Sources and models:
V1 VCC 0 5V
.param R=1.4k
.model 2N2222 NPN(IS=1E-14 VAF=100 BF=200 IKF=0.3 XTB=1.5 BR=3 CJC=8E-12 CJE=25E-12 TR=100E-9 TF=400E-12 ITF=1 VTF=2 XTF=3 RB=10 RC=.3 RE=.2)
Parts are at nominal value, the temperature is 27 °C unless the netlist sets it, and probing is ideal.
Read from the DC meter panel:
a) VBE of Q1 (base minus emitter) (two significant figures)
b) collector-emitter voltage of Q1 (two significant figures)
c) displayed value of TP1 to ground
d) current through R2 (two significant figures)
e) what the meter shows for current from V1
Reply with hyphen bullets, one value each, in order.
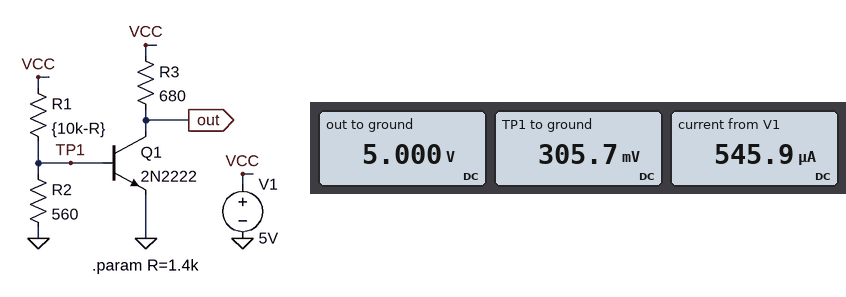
- 310 mV
- 5.0 V
- 305.7 mV
- 550 µA
- 545.9 µA
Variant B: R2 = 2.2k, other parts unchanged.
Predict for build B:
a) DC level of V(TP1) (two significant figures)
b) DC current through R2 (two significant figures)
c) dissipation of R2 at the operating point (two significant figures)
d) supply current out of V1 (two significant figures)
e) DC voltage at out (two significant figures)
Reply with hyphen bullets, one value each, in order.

- 710 mV
- 320 µA
- 230 µW
- 7.7 mA
- 81 mV
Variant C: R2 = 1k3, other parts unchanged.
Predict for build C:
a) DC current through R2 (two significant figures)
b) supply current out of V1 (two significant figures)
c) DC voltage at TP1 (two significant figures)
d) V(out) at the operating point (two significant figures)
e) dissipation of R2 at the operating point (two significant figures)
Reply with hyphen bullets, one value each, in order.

- 500 µA
- 1.4 mA
- 650 mV
- 4.4 V
- 330 µW
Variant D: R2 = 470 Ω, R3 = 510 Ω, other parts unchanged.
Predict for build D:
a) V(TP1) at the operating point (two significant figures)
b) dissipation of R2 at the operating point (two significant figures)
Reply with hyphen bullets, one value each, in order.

- 260 mV
- 140 µW
